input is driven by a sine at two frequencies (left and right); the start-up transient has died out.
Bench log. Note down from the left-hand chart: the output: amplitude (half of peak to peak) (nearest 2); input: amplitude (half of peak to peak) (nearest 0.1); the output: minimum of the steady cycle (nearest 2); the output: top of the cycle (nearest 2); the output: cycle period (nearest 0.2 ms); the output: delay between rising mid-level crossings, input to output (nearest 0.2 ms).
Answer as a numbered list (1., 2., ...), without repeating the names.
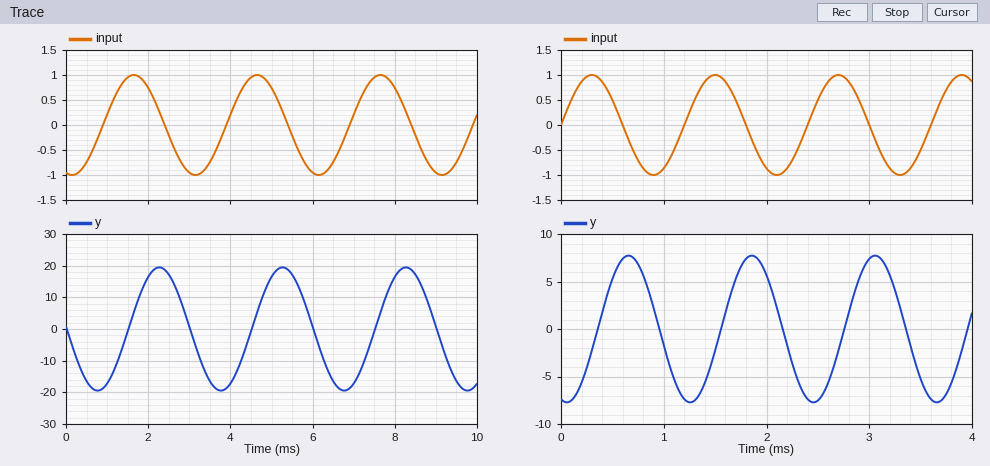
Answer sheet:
1. 20
2. 1.0
3. -20
4. 20
5. 3.0 ms
6. 0.6 ms
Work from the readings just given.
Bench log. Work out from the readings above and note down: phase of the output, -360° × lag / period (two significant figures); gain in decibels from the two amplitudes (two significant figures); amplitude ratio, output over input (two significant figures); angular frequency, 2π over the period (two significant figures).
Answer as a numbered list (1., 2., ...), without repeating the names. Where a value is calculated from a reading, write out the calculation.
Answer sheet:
1. -360 × 0.6 / 3 = -72°
2. 20 log10(20 / 1) = 26 dB
3. 20 / 1 = 20
4. 2π / 3 = 2.1 rad/ms
